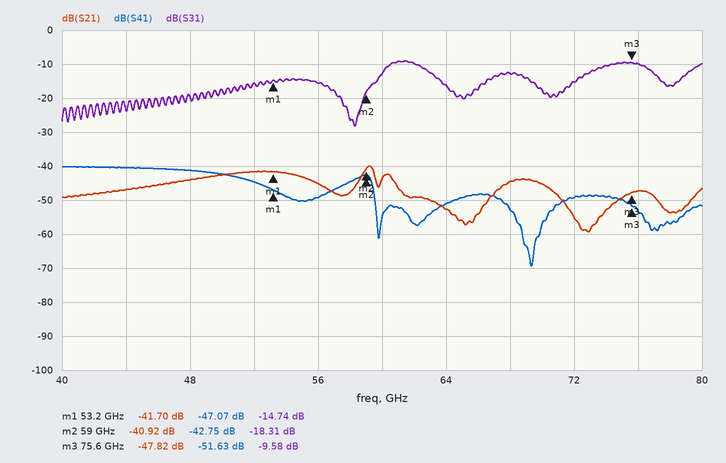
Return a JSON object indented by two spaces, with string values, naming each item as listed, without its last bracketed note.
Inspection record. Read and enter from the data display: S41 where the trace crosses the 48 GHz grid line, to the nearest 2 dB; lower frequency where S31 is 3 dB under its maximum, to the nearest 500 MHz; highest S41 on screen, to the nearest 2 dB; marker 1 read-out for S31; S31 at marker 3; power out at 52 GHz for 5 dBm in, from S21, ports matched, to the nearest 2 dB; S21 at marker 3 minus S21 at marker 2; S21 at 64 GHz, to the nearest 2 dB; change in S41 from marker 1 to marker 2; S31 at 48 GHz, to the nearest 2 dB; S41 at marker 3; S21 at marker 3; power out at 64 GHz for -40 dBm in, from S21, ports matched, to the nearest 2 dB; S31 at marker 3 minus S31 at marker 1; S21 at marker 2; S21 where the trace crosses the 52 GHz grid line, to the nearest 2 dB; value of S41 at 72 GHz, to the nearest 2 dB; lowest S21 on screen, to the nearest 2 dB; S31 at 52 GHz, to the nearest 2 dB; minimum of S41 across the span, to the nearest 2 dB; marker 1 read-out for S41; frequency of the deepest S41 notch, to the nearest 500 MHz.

{
  "S41 where the trace crosses the 48 GHz grid line, to the nearest 2 dB": "-42 dB",
  "lower frequency where S31 is 3 dB under its maximum, to the nearest 500 MHz": "60.0 GHz",
  "highest S41 on screen, to the nearest 2 dB": "-40 dB",
  "marker 1 read-out for S31": "-14.74 dB",
  "S31 at marker 3": "-9.58 dB",
  "power out at 52 GHz for 5 dBm in, from S21, ports matched, to the nearest 2 dB": "-36 dBm",
  "S21 at marker 3 minus S21 at marker 2": "-6.90 dB",
  "S21 at 64 GHz, to the nearest 2 dB": "-52 dB",
  "change in S41 from marker 1 to marker 2": "4.32 dB",
  "S31 at 48 GHz, to the nearest 2 dB": "-20 dB",
  "S41 at marker 3": "-51.63 dB",
  "S21 at marker 3": "-47.82 dB",
  "power out at 64 GHz for -40 dBm in, from S21, ports matched, to the nearest 2 dB": "-92 dBm",
  "S31 at marker 3 minus S31 at marker 1": "5.16 dB",
  "S21 at marker 2": "-40.92 dB",
  "S21 where the trace crosses the 52 GHz grid line, to the nearest 2 dB": "-42 dB",
  "value of S41 at 72 GHz, to the nearest 2 dB": "-50 dB",
  "lowest S21 on screen, to the nearest 2 dB": "-60 dB",
  "S31 at 52 GHz, to the nearest 2 dB": "-16 dB",
  "minimum of S41 across the span, to the nearest 2 dB": "-70 dB",
  "marker 1 read-out for S41": "-47.07 dB",
  "frequency of the deepest S41 notch, to the nearest 500 MHz": "69.5 GHz"
}
